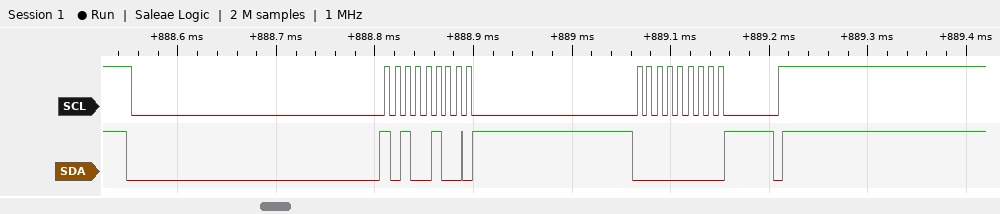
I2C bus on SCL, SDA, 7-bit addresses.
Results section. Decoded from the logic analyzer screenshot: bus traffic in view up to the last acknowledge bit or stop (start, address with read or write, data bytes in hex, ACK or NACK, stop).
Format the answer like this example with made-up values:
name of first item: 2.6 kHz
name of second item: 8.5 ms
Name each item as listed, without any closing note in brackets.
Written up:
bus traffic in view up to the last acknowledge bit or stop: start, address 52 write ACK, 00 ACK, stop
